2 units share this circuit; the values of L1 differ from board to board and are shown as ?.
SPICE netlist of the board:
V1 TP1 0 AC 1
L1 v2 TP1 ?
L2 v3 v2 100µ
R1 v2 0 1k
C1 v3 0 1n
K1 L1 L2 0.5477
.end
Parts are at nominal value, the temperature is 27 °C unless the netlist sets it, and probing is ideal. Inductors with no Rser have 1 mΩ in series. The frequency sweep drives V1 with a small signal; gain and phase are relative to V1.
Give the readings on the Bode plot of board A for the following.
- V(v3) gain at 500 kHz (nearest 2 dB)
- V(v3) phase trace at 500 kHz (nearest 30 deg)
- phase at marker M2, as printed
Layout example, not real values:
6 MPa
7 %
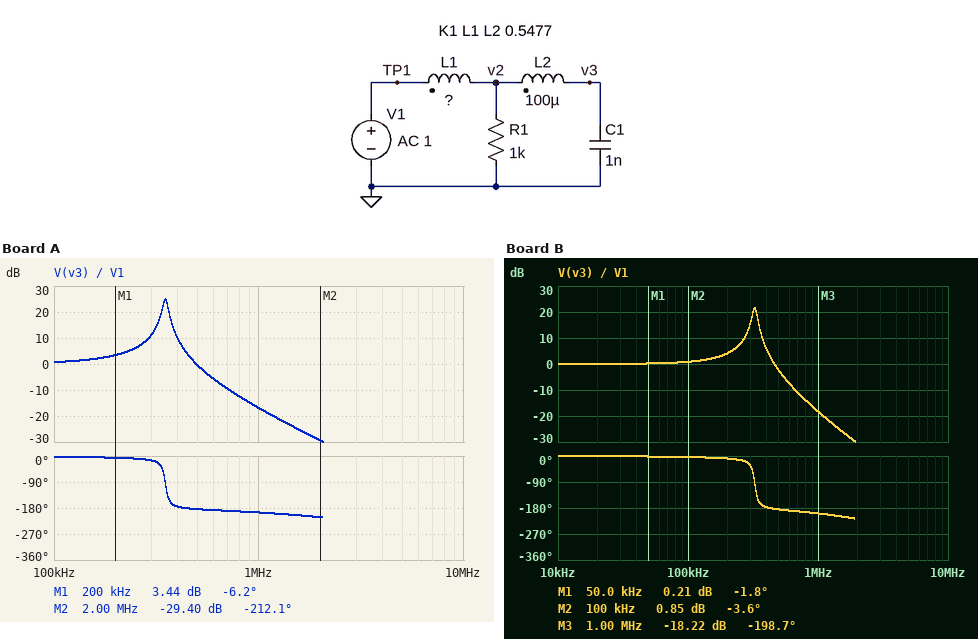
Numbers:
0 dB
-180 deg
-212.1 deg
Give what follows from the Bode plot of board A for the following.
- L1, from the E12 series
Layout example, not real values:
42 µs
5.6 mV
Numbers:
39 µH
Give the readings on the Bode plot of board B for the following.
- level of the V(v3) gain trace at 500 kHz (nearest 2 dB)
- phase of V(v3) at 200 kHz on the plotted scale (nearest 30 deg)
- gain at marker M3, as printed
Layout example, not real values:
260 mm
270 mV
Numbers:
-2 dB
0 deg
-18.22 dB
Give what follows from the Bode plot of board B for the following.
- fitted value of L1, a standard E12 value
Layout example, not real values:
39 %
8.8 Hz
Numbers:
56 µH
